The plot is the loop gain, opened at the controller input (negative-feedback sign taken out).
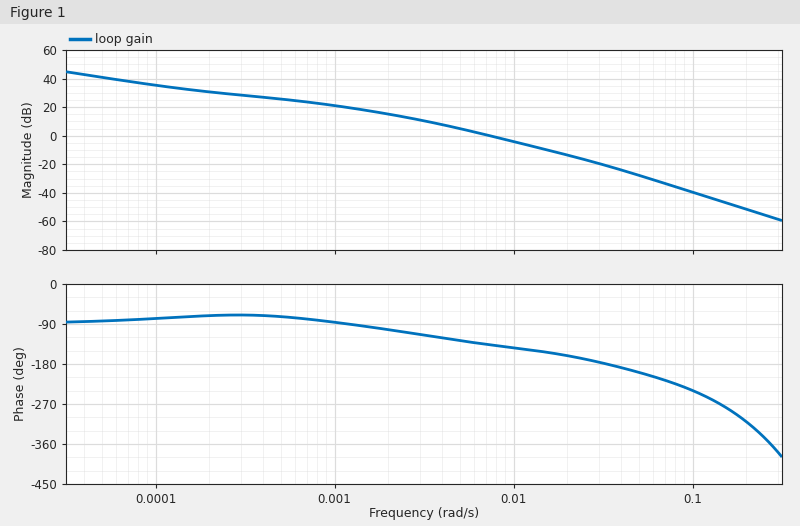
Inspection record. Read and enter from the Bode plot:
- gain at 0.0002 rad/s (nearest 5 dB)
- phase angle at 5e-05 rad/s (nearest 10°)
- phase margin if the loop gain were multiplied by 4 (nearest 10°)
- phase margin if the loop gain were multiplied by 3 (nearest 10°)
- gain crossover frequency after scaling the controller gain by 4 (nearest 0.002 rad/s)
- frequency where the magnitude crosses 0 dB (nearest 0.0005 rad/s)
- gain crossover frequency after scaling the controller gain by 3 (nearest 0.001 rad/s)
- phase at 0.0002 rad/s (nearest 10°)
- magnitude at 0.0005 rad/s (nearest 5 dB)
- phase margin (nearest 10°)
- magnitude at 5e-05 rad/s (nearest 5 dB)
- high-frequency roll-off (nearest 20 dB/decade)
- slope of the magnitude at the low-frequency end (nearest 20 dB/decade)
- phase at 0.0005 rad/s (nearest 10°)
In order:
30 dB
-80°
20°
30°
0.018 rad/s
0.0075 rad/s
0.015 rad/s
-70°
25 dB
40°
40 dB
-40 dB/decade
-20 dB/decade
-70°
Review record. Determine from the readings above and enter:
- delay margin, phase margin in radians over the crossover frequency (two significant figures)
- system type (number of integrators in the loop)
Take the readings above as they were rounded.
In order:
93 s
1
